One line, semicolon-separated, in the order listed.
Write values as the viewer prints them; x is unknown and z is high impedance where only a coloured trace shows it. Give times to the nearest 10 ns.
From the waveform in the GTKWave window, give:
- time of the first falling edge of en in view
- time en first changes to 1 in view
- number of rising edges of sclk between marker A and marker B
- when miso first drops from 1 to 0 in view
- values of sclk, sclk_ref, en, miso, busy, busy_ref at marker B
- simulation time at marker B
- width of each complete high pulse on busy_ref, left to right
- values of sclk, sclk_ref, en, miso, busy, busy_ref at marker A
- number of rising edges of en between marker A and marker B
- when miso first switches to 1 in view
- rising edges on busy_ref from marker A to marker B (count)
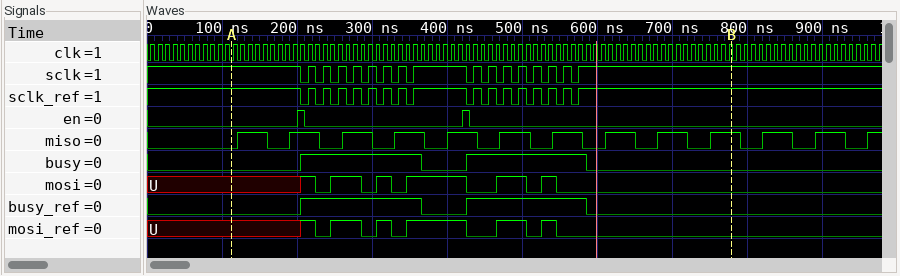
210 ns; 200 ns; 16; 160 ns; sclk=1, sclk_ref=1, en=0, miso=1, busy=0, busy_ref=0; 780 ns; 160 ns, 160 ns; sclk=1, sclk_ref=1, en=0, miso=0, busy=0, busy_ref=0; 2; 120 ns; 2
